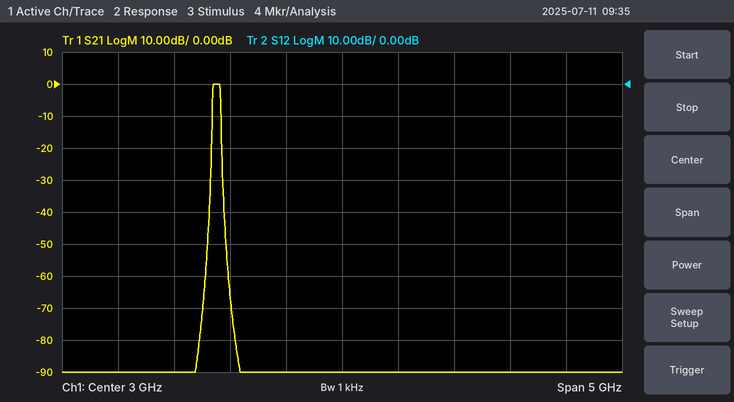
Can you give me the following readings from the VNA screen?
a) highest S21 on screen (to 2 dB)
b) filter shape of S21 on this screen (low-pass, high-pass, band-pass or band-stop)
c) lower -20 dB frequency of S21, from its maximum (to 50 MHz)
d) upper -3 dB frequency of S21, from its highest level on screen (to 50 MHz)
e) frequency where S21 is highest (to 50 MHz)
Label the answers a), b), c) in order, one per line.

a) 0 dB
b) band-pass
c) 1.85 GHz
d) 1.90 GHz
e) 1.85 GHz
